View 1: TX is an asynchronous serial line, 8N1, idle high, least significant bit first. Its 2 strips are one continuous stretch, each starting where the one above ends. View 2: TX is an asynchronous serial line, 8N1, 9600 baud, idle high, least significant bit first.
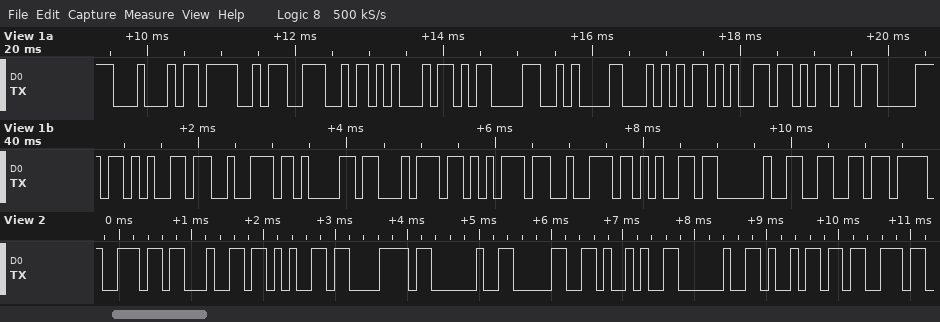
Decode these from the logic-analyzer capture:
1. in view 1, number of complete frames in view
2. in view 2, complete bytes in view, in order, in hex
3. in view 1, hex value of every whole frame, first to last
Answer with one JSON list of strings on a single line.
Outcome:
["19", "6E 64 65 78 20 30 29 20 69 73", "0x44 0x4F 0x4E 0x45 0x0D 0x0A 0x54 0x65 0x6D 0x70 0x65 0x72 0x61 0x74 0x75 0x72 0x65 0x20 0x66"]
